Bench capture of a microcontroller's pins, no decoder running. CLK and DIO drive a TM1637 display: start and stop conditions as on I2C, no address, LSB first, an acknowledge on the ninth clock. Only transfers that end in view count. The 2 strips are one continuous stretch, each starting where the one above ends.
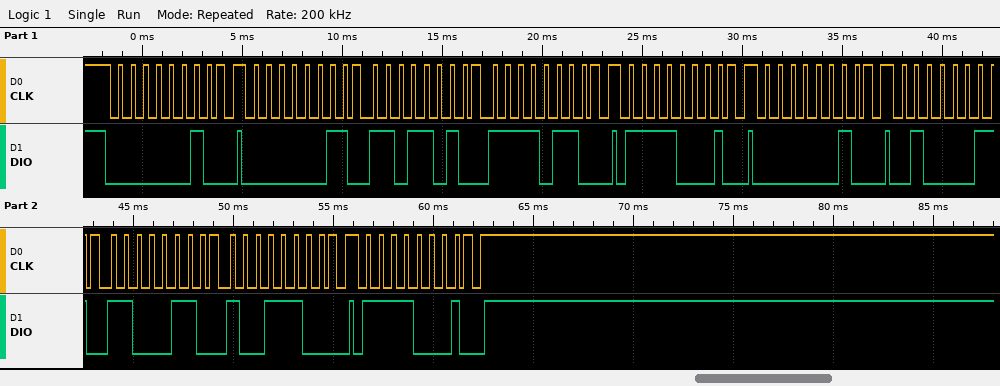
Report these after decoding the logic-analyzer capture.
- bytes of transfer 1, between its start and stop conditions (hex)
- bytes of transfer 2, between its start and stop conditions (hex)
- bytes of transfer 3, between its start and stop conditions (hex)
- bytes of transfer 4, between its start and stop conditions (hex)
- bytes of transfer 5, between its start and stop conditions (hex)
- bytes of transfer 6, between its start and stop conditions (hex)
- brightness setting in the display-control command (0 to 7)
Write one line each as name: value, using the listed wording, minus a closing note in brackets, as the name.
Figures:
bytes of transfer 1, between its start and stop conditions: 40
bytes of transfer 2, between its start and stop conditions: C0 5B 6F
bytes of transfer 3, between its start and stop conditions: 8F
bytes of transfer 4, between its start and stop conditions: 40
bytes of transfer 5, between its start and stop conditions: C2 63 39
bytes of transfer 6, between its start and stop conditions: 8F
brightness setting in the display-control command: 7
